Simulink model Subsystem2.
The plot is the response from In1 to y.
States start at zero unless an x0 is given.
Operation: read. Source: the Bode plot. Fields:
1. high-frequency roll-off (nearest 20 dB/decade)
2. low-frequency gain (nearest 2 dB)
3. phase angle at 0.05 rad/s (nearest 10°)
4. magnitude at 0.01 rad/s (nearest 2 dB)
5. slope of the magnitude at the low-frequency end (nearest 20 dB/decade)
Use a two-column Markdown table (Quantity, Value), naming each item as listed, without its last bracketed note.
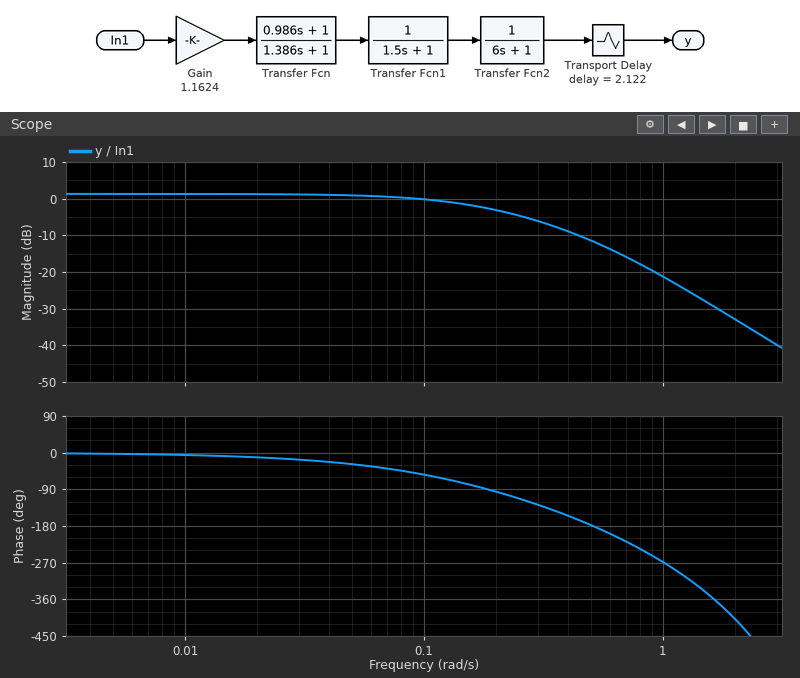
| Quantity | Value |
|---|---|
| high-frequency roll-off | -40 dB/decade |
| low-frequency gain | 2 dB |
| phase angle at 0.05 rad/s | -30° |
| magnitude at 0.01 rad/s | 2 dB |
| slope of the magnitude at the low-frequency end | 0 dB/decade |
